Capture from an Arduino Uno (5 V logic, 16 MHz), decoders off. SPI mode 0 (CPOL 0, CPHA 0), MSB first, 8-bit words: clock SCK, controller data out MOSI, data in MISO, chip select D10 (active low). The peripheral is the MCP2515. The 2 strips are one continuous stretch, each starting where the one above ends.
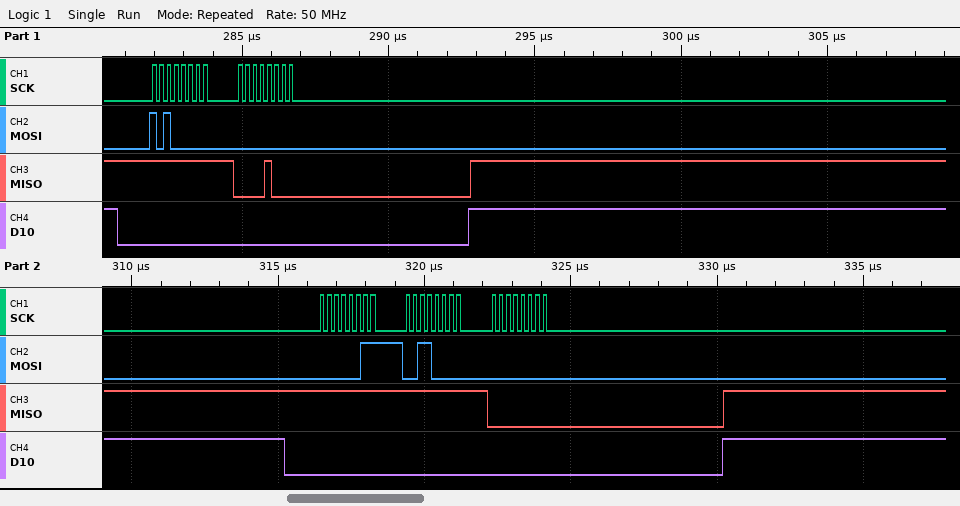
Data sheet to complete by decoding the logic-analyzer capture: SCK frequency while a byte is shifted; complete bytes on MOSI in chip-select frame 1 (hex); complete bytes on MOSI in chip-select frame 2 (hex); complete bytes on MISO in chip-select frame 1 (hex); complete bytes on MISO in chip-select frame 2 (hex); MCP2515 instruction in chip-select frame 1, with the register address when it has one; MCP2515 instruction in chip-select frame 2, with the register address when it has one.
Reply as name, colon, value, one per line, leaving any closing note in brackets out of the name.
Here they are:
SCK frequency while a byte is shifted: 4 MHz
complete bytes on MOSI in chip-select frame 1: A0 00
complete bytes on MOSI in chip-select frame 2: 03 30 00
complete bytes on MISO in chip-select frame 1: FF 08
complete bytes on MISO in chip-select frame 2: FF FF 00
MCP2515 instruction in chip-select frame 1, with the register address when it has one: READ STATUS
MCP2515 instruction in chip-select frame 2, with the register address when it has one: READ 0x30
